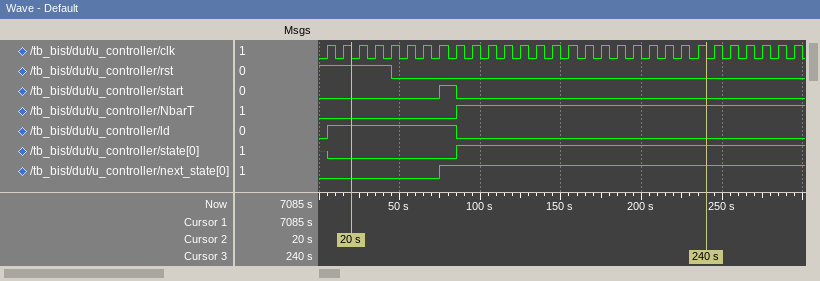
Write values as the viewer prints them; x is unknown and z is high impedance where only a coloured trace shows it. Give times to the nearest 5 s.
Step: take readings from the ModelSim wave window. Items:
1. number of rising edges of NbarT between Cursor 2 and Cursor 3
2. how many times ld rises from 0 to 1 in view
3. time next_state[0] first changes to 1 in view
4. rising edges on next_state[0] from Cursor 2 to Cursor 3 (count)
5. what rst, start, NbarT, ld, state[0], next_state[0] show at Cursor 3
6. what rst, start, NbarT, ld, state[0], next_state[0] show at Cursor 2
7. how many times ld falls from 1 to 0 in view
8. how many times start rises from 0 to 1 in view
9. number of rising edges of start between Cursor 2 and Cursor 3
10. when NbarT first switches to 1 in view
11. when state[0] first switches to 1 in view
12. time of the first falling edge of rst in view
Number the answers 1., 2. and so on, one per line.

1. 1
2. 1
3. 75 s
4. 1
5. rst=0, start=0, NbarT=1, ld=0, state[0]=1, next_state[0]=1
6. rst=1, start=0, NbarT=0, ld=1, state[0]=0, next_state[0]=0
7. 1
8. 1
9. 1
10. 85 s
11. 85 s
12. 45 s
